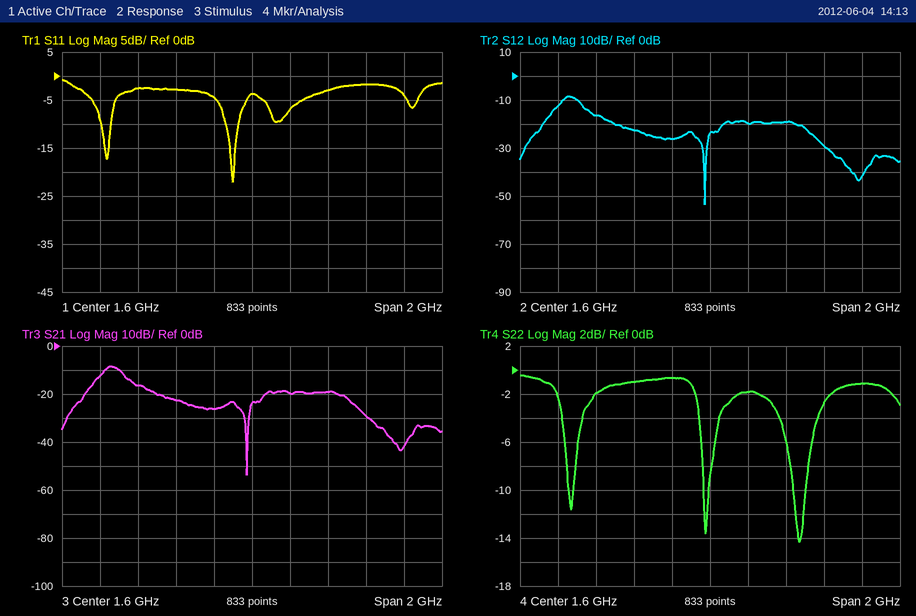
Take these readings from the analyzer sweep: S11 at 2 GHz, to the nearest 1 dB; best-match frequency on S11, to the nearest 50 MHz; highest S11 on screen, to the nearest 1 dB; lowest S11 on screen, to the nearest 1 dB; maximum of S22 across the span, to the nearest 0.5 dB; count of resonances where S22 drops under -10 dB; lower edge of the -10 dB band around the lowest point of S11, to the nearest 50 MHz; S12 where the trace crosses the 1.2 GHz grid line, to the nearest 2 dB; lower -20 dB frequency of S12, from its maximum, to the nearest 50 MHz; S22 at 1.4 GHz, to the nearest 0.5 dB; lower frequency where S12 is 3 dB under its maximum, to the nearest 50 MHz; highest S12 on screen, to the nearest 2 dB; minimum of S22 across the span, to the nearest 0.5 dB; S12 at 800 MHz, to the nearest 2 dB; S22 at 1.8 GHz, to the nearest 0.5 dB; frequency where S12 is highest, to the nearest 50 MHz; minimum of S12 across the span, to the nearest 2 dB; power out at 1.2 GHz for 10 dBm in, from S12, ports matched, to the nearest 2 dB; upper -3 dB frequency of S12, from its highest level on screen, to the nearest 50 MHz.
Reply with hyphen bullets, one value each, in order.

- -3 dB
- 1.50 GHz
- -1 dB
- -22 dB
- -0.5 dB
- 3
- 1.45 GHz
- -22 dB
- 650 MHz
- -0.5 dB
- 800 MHz
- -8 dB
- -14.5 dB
- -12 dB
- -2.0 dB
- 850 MHz
- -54 dB
- -12 dBm
- 900 MHz
